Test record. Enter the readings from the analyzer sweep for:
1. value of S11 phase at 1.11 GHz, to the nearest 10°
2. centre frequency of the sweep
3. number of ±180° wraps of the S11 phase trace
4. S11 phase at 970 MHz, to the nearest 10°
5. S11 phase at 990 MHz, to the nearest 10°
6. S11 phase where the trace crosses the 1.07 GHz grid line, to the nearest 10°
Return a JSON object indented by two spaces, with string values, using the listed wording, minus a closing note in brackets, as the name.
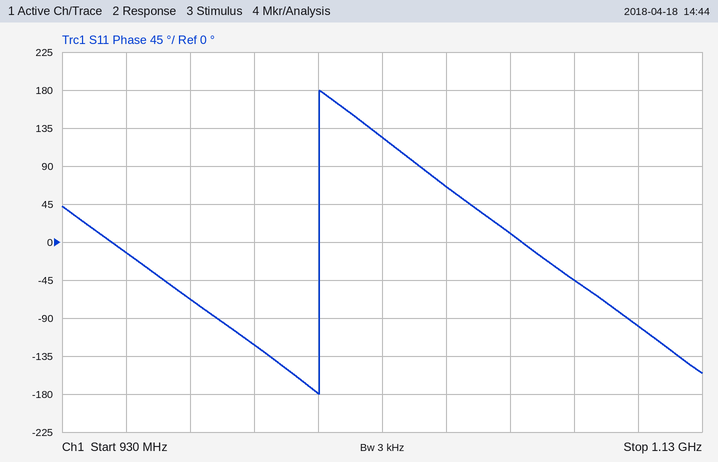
{
  "value of S11 phase at 1.11 GHz, to the nearest 10°": "-100°",
  "centre frequency of the sweep": "1.03 GHz",
  "number of ±180° wraps of the S11 phase trace": "1",
  "S11 phase at 970 MHz, to the nearest 10°": "-70°",
  "S11 phase at 990 MHz, to the nearest 10°": "-120°",
  "S11 phase where the trace crosses the 1.07 GHz grid line, to the nearest 10°": "10°"
}
